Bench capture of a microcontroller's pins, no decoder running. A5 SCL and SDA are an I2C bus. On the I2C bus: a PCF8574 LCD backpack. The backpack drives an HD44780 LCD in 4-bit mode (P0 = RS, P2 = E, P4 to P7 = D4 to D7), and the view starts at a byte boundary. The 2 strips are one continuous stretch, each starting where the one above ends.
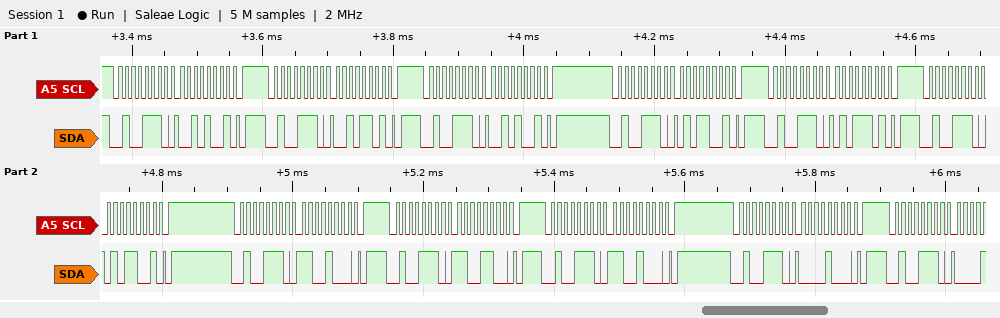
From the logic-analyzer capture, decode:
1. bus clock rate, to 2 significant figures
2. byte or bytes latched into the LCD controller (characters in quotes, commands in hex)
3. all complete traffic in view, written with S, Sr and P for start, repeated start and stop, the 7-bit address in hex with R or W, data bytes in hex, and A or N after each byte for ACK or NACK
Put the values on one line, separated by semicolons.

100 kHz; '%'; S 27W A 29 A P S 27W A 2D A P S 27W A 29 A P S 27W A 59 A P S 27W A 5D A P S 27W A 59 A P S 27W A C8 A P S 27W A CC A P S 27W A C8 A P S 27W A 08 A P S 27W A
